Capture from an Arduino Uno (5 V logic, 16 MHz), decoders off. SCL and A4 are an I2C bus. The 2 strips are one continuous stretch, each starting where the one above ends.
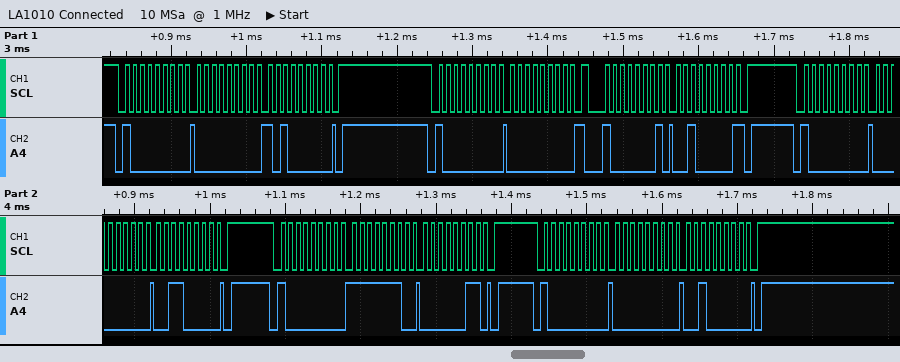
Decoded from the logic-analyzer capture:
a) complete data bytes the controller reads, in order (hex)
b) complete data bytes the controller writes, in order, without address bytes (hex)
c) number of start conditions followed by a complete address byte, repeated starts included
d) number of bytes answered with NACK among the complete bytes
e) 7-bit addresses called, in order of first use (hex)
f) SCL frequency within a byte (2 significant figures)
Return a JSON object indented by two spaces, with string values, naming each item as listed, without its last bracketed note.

{
  "complete data bytes the controller reads, in order": "20",
  "complete data bytes the controller writes, in order, without address bytes": "00 A0 00 00 30 FE 03 00 20",
  "number of start conditions followed by a complete address byte, repeated starts included": "6",
  "number of bytes answered with NACK among the complete bytes": "1",
  "7-bit addresses called, in order of first use": "0x40",
  "SCL frequency within a byte": "100 kHz"
}
